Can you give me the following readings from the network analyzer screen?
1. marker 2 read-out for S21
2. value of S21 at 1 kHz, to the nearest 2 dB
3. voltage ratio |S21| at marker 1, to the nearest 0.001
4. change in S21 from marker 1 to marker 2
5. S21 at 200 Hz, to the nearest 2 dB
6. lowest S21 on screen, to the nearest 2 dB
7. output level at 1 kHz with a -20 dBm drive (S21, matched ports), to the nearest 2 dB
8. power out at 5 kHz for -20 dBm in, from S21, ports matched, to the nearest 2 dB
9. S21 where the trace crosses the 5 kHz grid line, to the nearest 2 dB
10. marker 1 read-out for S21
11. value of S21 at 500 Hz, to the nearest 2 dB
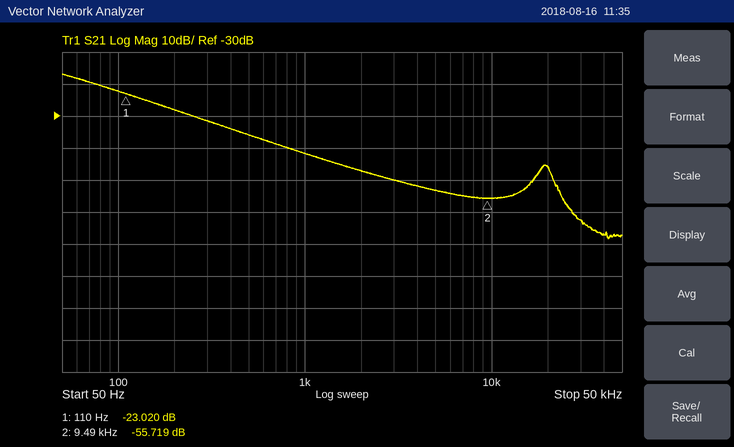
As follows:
-55.719 dB
-42 dB
0.071
-32.699 dB
-28 dB
-68 dB
-62 dBm
-74 dBm
-54 dB
-23.020 dB
-36 dB
